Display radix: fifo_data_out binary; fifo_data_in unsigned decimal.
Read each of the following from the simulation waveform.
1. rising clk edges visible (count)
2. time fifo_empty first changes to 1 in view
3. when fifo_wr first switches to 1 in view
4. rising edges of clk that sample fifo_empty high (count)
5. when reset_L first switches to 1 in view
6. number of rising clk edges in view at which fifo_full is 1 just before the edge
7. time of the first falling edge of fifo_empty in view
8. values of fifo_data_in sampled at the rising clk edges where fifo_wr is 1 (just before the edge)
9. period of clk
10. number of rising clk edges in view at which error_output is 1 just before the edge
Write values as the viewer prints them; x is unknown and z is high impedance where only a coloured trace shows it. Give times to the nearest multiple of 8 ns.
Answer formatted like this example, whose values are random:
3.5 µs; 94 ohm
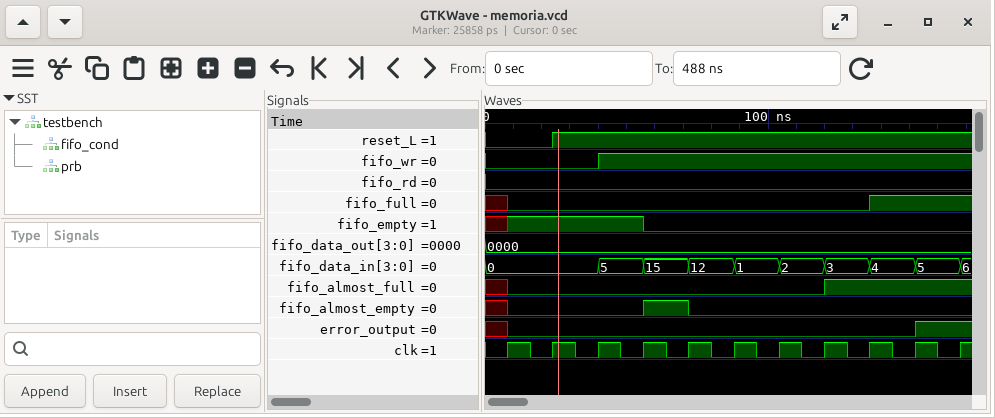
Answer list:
11; 8 ns; 40 ns; 3; 24 ns; 2; 56 ns; 5, 15, 12, 1, 2, 3, 4, 5; 16 ns; 1
